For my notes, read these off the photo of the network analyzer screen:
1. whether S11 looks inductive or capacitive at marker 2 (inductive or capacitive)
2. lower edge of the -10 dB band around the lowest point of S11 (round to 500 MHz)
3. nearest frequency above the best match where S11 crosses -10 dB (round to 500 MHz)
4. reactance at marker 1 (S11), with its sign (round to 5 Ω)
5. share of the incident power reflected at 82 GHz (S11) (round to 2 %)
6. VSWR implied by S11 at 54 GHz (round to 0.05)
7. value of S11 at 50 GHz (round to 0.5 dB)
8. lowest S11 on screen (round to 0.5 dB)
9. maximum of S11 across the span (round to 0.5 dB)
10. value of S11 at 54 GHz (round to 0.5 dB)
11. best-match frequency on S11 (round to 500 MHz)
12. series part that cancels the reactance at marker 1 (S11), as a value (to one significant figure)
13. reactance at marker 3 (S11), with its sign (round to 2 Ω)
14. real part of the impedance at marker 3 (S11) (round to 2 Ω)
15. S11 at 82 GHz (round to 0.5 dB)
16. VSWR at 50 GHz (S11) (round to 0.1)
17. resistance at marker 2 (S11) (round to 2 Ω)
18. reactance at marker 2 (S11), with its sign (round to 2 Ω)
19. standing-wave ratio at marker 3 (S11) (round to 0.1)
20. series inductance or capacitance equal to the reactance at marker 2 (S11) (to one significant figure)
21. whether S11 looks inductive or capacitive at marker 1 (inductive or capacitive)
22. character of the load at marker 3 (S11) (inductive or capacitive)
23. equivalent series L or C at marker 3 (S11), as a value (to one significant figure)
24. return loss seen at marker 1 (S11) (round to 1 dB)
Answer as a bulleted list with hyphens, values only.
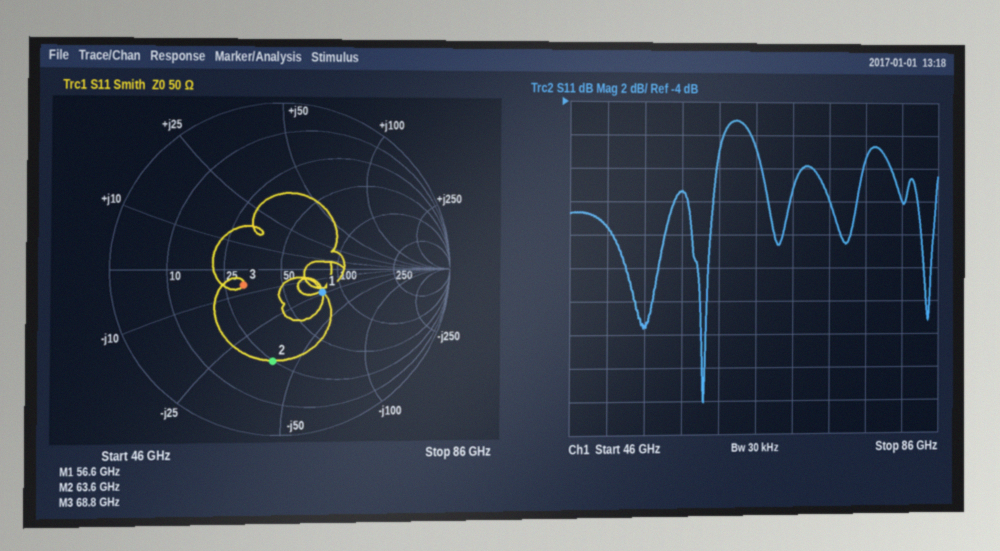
- capacitive
- 58.5 GHz
- 61.5 GHz
- -25 Ω
- 10 %
- 1.30
- -11.5 dB
- -22.0 dB
- -5.0 dB
- -17.5 dB
- 60.5 GHz
- 70 pH
- -6 Ω
- 32 Ω
- -10.0 dB
- 1.7
- 24 Ω
- -40 Ω
- 1.6
- 60 fF
- capacitive
- capacitive
- 400 fF
- 11 dB
